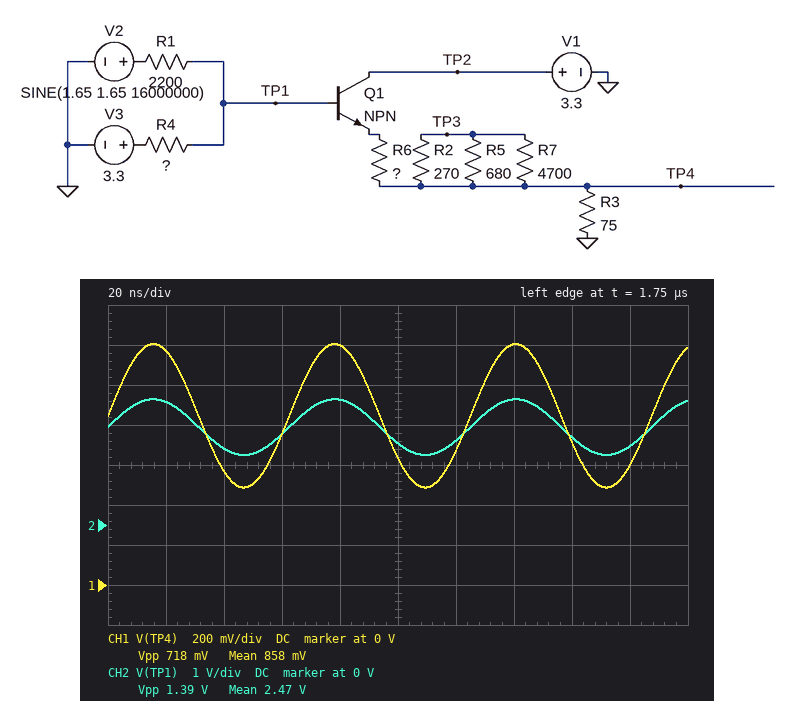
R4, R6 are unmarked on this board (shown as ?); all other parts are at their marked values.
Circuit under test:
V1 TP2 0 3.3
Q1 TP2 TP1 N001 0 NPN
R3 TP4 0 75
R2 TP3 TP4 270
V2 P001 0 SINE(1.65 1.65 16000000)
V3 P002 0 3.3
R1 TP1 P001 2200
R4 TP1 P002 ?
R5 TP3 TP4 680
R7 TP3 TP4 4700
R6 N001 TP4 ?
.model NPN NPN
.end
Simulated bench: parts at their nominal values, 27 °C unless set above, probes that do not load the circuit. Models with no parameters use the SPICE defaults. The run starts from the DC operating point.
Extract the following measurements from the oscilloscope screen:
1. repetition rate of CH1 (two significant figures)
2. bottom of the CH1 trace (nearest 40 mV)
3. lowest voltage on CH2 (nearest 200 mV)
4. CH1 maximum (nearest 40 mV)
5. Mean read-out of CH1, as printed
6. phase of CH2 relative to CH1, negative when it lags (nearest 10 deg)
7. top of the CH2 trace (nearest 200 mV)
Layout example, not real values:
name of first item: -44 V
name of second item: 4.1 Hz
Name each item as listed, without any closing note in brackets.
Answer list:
repetition rate of CH1: 16 MHz
bottom of the CH1 trace: 480 mV
lowest voltage on CH2: 1.8 V
CH1 maximum: 1.20 V
Mean read-out of CH1, as printed: 858 mV
phase of CH2 relative to CH1, negative when it lags: 0 deg
top of the CH2 trace: 3.2 V
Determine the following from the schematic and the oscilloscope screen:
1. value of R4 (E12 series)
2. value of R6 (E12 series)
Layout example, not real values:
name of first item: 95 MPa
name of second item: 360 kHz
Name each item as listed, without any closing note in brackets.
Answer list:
value of R4: 1.8 kΩ
value of R6: 68 Ω
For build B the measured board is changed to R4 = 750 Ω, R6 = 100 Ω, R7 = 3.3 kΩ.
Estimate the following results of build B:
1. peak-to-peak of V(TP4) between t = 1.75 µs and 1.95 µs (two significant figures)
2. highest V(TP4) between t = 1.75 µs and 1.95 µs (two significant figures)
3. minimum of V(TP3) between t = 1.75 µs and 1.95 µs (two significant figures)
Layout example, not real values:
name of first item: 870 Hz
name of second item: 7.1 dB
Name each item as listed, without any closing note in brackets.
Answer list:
peak-to-peak of V(TP4) between t = 1.75 µs and 1.95 µs: 340 mV
highest V(TP4) between t = 1.75 µs and 1.95 µs: 1.0 V
minimum of V(TP3) between t = 1.75 µs and 1.95 µs: 680 mV
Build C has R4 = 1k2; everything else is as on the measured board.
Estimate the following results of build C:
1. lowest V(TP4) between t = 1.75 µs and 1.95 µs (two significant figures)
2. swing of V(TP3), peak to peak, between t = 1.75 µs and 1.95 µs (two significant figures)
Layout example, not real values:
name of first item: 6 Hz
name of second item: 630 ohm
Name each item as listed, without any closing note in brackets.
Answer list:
lowest V(TP4) between t = 1.75 µs and 1.95 µs: 650 mV
swing of V(TP3), peak to peak, between t = 1.75 µs and 1.95 µs: 570 mV
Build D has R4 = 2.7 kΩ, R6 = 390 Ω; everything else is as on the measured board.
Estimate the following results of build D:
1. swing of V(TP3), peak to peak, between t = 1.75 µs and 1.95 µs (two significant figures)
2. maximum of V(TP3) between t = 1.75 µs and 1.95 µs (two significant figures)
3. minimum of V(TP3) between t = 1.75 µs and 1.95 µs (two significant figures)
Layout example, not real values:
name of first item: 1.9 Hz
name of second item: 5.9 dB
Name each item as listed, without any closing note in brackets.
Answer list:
swing of V(TP3), peak to peak, between t = 1.75 µs and 1.95 µs: 280 mV
maximum of V(TP3) between t = 1.75 µs and 1.95 µs: 390 mV
minimum of V(TP3) between t = 1.75 µs and 1.95 µs: 110 mV
